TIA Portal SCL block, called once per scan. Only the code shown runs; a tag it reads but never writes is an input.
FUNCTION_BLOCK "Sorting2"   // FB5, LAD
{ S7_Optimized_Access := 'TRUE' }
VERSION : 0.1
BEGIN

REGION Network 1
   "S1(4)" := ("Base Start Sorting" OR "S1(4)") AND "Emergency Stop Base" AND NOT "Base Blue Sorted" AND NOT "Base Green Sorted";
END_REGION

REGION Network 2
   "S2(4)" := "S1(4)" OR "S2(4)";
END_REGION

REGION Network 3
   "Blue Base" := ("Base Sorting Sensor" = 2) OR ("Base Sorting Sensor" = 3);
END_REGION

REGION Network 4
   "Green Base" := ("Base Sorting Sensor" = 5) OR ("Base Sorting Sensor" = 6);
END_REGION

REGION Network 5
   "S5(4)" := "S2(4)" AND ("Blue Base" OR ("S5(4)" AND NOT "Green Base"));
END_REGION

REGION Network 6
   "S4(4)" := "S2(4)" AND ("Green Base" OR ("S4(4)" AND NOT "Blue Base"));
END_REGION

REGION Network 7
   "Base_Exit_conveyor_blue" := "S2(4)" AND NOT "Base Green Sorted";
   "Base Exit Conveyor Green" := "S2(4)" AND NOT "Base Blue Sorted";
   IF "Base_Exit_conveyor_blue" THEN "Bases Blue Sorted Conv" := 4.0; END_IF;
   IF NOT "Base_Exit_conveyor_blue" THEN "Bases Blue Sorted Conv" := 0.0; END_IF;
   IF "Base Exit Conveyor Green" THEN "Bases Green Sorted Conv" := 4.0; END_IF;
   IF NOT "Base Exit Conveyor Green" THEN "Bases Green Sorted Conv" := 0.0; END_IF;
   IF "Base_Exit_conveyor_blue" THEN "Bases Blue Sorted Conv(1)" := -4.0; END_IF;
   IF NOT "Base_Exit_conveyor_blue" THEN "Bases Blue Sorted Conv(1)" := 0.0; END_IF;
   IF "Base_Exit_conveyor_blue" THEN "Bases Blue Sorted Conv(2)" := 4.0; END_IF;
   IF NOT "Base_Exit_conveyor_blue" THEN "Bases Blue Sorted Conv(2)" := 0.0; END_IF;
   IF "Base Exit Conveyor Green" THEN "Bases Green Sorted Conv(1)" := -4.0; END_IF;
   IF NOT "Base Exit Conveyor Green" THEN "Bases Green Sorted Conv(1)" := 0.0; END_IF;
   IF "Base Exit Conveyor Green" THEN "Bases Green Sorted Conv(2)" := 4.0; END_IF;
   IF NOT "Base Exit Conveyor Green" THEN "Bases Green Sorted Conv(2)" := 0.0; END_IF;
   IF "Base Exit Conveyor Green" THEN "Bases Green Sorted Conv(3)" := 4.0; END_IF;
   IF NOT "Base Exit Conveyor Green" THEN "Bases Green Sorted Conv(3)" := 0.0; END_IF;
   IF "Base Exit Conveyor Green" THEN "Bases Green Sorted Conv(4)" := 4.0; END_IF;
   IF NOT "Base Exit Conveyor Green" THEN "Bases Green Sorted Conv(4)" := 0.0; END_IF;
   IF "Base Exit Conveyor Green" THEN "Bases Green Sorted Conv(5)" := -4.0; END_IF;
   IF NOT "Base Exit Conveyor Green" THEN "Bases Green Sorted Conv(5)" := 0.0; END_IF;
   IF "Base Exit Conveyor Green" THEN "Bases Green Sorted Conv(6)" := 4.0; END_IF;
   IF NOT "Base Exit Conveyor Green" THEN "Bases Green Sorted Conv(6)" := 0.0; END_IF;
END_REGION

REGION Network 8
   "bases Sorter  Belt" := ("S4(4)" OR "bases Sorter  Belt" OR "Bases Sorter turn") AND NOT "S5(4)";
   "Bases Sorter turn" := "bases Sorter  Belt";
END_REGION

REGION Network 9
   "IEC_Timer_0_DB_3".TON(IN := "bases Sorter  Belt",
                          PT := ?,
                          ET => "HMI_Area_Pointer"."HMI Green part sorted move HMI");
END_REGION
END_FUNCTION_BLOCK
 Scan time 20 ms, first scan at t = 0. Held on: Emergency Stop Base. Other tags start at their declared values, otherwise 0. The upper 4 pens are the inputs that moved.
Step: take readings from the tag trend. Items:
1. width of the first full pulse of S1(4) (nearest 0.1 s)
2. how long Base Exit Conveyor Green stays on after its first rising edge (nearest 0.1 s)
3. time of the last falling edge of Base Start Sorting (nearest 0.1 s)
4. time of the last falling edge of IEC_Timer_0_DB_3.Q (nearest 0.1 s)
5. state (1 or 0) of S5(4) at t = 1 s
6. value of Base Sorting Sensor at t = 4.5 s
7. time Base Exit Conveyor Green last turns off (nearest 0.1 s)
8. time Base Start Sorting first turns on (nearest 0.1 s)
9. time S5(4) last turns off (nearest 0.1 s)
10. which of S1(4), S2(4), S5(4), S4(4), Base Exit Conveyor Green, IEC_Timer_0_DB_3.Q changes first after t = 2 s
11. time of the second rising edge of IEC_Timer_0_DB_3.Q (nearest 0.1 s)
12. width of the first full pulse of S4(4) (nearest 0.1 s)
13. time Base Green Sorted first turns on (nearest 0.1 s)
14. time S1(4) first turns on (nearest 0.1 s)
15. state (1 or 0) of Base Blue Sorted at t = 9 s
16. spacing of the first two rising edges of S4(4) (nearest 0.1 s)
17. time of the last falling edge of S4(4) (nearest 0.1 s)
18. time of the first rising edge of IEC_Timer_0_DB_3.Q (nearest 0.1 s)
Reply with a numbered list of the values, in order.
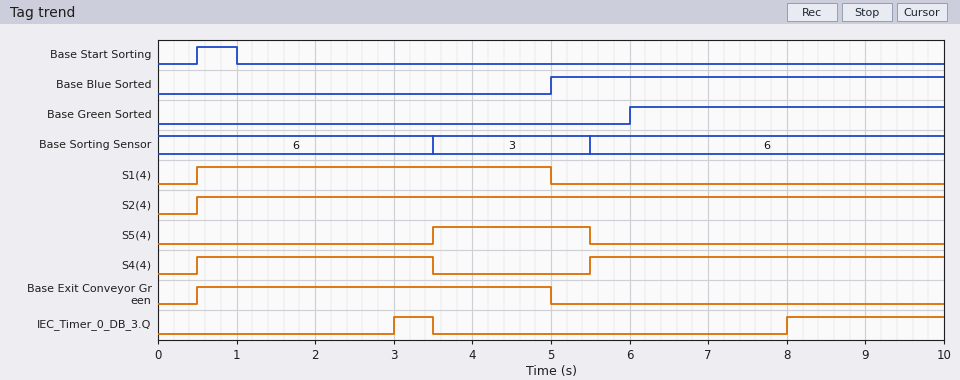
1. 4.5 s
2. 4.5 s
3. 1.0 s
4. 3.5 s
5. 0
6. 3
7. 5.0 s
8. 0.5 s
9. 5.5 s
10. IEC_Timer_0_DB_3.Q
11. 8.0 s
12. 3.0 s
13. 6.0 s
14. 0.5 s
15. 1
16. 5.0 s
17. 3.5 s
18. 3.0 s
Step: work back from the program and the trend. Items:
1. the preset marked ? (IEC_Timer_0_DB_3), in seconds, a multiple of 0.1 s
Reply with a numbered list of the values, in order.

1. 2.5 s
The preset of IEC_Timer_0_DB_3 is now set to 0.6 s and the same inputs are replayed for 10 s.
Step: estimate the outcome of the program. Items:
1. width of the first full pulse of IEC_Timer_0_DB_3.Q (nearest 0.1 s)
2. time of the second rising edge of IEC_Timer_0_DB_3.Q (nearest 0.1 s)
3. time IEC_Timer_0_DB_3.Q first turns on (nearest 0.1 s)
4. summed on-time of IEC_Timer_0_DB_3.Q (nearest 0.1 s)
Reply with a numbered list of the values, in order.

1. 2.4 s
2. 6.1 s
3. 1.1 s
4. 6.3 s
